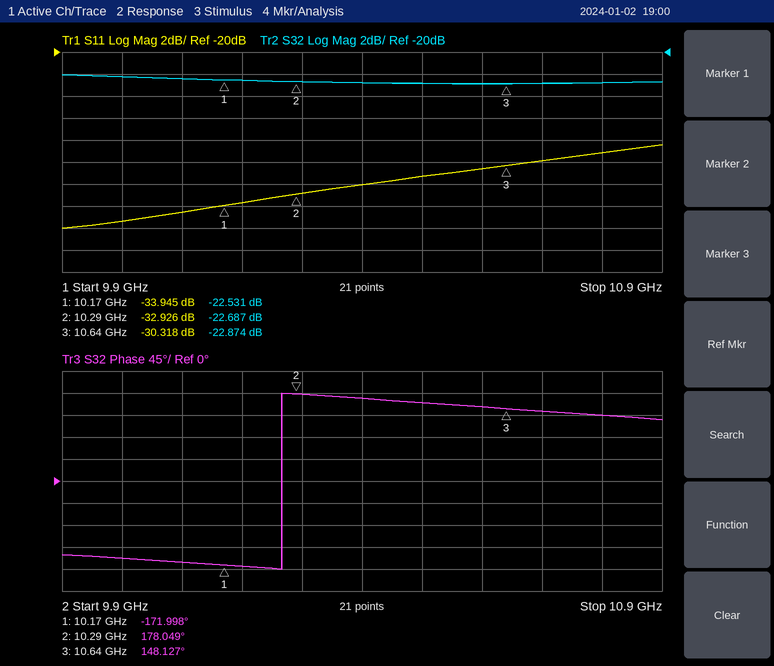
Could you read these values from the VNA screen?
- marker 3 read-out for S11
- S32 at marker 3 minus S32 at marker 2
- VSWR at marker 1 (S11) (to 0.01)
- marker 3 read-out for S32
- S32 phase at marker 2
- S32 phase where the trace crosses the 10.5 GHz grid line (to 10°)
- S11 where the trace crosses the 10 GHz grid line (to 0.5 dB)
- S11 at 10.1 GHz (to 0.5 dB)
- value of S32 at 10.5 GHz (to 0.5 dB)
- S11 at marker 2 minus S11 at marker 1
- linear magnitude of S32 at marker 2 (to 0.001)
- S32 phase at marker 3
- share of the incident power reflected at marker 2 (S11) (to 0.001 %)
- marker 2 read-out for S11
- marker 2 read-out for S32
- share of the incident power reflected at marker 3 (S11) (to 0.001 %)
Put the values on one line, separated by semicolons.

-30.318 dB; -0.187 dB; 1.04; -22.874 dB; 178.049°; 160°; -35.5 dB; -34.5 dB; -23.0 dB; 1.019 dB; 0.073; 148.127°; 0.051 %; -32.926 dB; -22.687 dB; 0.093 %
